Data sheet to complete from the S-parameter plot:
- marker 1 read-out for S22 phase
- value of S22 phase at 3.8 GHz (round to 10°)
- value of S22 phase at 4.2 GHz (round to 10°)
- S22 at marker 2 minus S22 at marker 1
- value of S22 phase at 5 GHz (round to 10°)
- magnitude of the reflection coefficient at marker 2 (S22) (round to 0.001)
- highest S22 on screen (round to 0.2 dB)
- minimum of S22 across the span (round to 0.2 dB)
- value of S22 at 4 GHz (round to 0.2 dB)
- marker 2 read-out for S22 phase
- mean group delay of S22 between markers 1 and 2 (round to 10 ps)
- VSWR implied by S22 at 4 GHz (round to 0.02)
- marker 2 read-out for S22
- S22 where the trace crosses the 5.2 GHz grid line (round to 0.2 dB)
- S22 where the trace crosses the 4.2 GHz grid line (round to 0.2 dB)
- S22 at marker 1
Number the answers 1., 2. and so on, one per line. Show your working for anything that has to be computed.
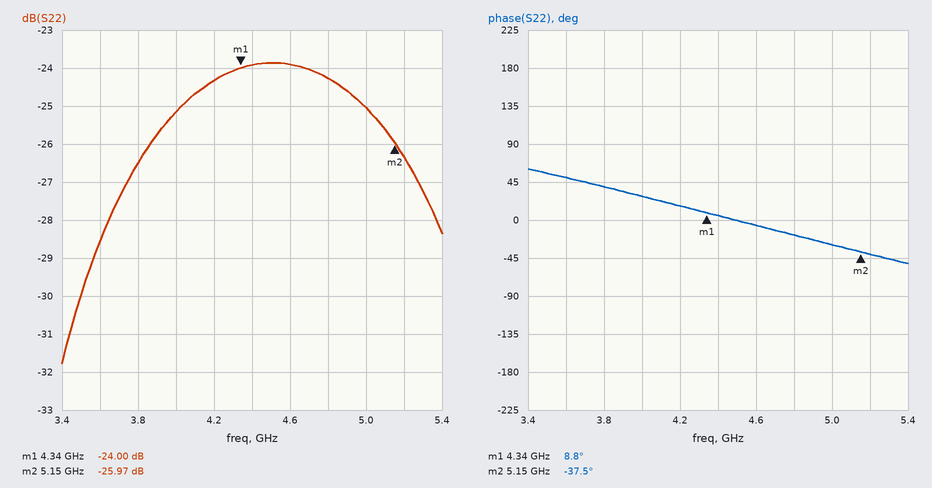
1. 8.8°
2. 40°
3. 20°
4. -25.97 − (-24) = -1.97 dB
5. -30°
6. 10^(-25.97/20) ≈ 0.050
7. -23.8 dB
8. -31.8 dB
9. -25.2 dB
10. -37.5°
11. −(-37.5° − (8.8°))/(360° × 810 MHz) ≈ 159 ps, so 160 ps to the nearest 10 ps
12. |Γ| = 10^(-25.2/20) = 0.0550; VSWR = (1 + 0.0550)/(1 − 0.0550) ≈ 1.12
13. -25.97 dB
14. -26.4 dB
15. -24.4 dB
16. -24.00 dB
